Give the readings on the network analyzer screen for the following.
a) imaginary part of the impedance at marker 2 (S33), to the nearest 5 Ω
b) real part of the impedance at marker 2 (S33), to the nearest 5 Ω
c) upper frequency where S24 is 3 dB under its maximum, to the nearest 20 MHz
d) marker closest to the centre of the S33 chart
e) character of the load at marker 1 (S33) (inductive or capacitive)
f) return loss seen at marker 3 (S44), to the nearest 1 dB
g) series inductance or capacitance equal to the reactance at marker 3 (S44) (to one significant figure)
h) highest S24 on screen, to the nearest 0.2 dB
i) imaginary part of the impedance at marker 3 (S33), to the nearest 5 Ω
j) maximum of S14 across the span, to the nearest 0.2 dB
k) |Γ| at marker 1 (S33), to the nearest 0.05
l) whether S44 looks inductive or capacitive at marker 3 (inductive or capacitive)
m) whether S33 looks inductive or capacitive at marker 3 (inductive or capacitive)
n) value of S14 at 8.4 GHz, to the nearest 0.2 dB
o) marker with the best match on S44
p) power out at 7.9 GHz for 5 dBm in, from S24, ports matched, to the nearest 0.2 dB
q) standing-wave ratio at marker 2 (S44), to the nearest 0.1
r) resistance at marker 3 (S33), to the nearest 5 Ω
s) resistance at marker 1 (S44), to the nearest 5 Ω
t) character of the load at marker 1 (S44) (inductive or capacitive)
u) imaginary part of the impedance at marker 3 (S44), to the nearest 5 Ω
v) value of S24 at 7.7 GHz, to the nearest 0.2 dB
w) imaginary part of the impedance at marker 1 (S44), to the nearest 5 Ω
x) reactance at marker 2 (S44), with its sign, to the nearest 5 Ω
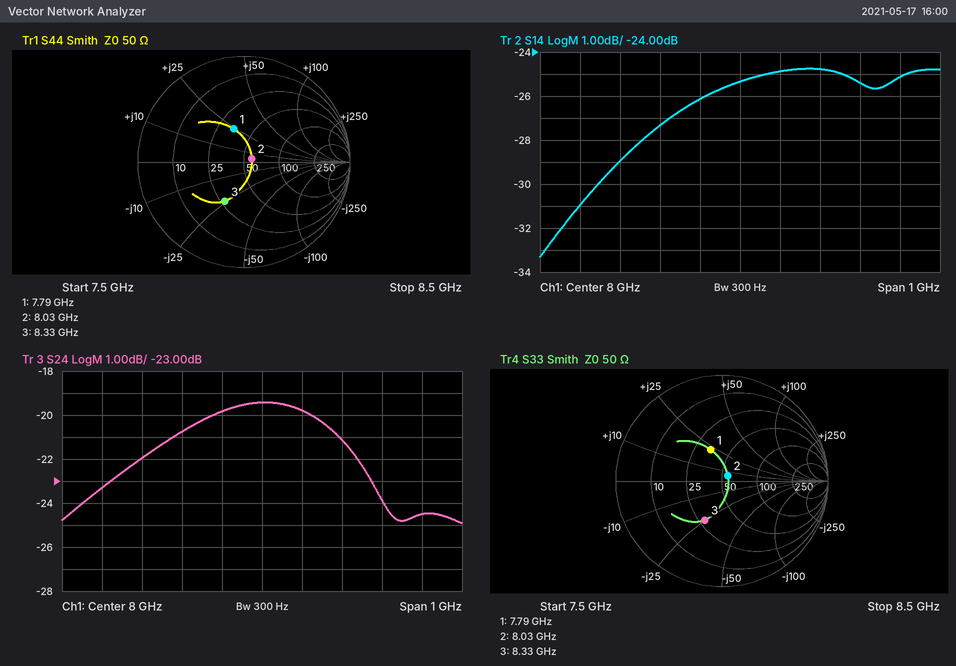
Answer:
+5 Ω
55 Ω
8.26 GHz
marker 2
inductive
8 dB
800 fF
-19.4 dB
-25 Ω
-24.8 dB
0.30
capacitive
capacitive
-25.2 dB
marker 2
-14.8 dBm
1.2
30 Ω
35 Ω
inductive
-25 Ω
-22.0 dB
+25 Ω
+5 Ω
